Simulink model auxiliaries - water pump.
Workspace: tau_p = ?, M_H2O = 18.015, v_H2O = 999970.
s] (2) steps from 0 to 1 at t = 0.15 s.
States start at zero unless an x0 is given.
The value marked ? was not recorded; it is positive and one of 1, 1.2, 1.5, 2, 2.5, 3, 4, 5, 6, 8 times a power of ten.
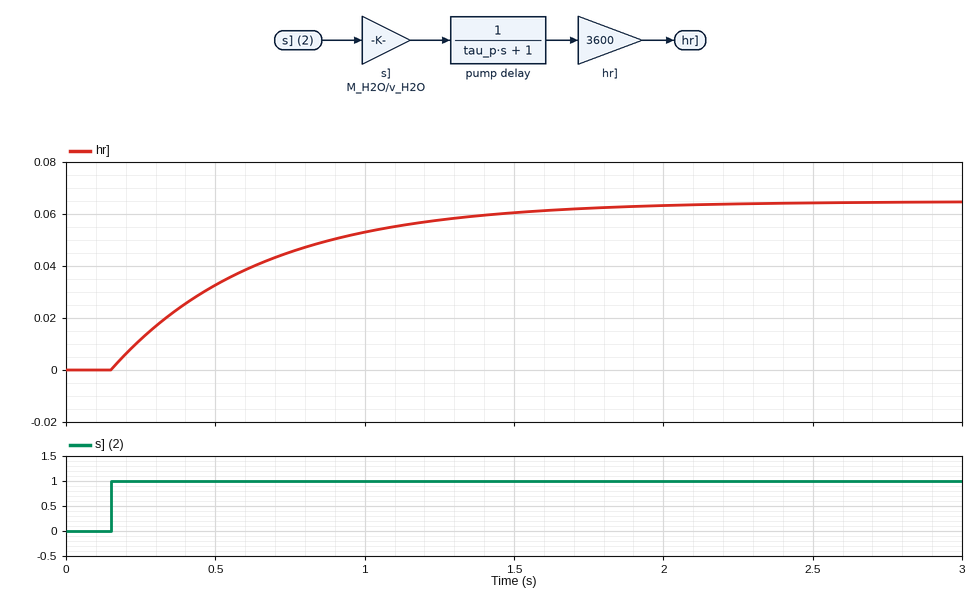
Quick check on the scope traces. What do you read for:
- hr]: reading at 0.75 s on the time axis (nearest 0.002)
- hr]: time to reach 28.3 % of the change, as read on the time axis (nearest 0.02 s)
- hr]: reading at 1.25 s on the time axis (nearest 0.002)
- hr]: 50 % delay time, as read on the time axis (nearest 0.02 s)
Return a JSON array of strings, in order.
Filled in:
["0.046", "0.32 s", "0.058", "0.50 s"]
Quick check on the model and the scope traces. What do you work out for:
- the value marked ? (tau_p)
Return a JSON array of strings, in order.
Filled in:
["0.5"]
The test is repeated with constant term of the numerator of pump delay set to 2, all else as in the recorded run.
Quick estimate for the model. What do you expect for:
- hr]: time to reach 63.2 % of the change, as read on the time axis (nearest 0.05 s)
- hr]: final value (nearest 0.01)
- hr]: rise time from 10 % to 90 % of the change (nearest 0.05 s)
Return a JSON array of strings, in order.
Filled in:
["0.65 s", "0.13", "1.10 s"]
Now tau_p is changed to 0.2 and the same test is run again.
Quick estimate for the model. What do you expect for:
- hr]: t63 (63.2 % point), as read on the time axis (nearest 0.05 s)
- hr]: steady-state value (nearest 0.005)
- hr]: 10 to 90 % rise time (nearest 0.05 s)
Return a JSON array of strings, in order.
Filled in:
["0.35 s", "0.065", "0.45 s"]
